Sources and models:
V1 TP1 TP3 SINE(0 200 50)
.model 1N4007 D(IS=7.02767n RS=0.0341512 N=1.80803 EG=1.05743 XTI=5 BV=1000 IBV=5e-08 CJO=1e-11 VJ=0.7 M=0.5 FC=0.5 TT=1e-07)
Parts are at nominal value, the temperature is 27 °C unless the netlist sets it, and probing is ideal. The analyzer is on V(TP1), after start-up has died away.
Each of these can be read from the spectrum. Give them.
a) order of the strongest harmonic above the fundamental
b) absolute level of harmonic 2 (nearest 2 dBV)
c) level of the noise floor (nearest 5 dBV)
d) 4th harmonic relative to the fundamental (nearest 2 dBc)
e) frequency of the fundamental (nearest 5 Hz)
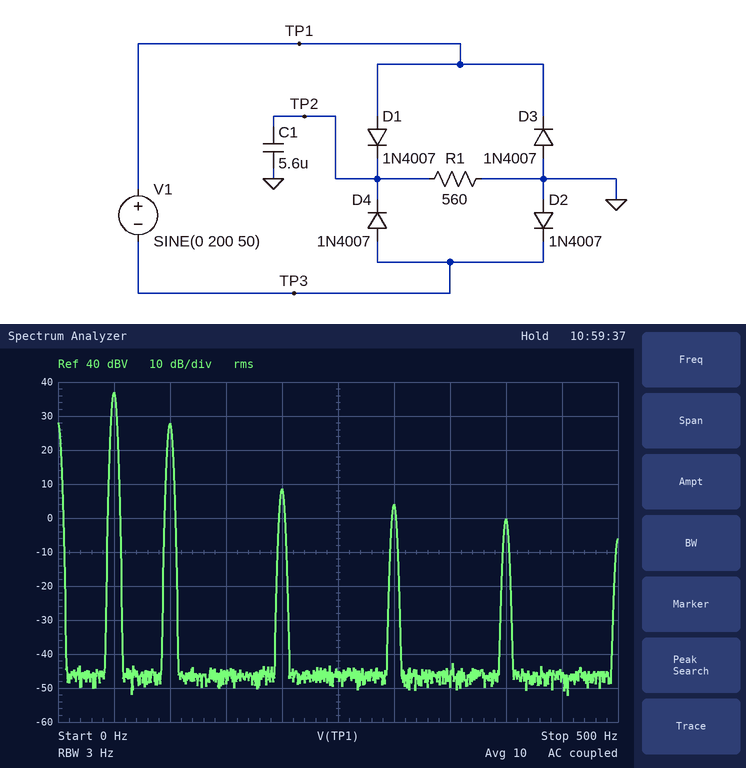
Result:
2
28 dBV
-45 dBV
-28 dBc
50 Hz
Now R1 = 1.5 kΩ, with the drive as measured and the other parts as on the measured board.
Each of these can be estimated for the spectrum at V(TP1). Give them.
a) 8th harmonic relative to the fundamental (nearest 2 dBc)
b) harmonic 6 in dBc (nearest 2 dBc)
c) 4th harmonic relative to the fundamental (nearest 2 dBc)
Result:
-38 dBc
-36 dBc
-26 dBc
